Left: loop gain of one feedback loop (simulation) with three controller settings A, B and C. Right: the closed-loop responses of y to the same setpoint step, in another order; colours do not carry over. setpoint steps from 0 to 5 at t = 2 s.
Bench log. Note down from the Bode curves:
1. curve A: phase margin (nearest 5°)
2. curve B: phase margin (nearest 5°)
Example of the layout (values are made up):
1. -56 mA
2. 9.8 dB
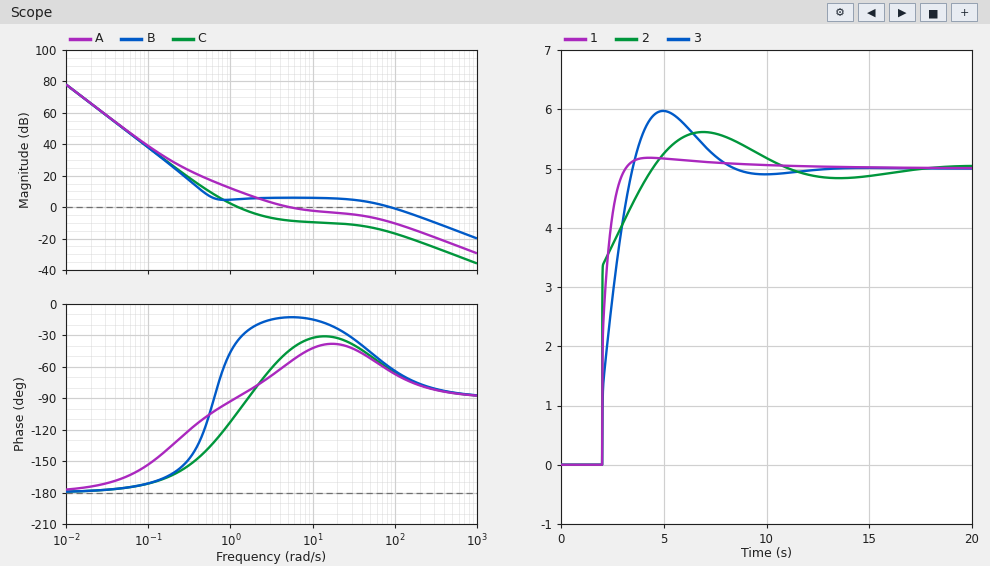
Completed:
1. 125°
2. 120°
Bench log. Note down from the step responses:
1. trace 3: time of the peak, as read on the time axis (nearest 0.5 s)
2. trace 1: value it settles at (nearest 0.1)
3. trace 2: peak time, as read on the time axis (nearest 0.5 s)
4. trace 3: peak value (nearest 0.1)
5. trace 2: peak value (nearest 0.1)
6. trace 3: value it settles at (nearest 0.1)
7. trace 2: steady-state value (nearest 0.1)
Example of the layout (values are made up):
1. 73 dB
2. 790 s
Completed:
1. 5.0 s
2. 5.0
3. 7.0 s
4. 6.0
5. 5.6
6. 5.0
7. 5.0
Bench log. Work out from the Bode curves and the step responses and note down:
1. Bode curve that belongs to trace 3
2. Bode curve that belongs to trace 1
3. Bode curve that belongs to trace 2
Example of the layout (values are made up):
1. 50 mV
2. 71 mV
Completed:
1. C
2. A
3. B
